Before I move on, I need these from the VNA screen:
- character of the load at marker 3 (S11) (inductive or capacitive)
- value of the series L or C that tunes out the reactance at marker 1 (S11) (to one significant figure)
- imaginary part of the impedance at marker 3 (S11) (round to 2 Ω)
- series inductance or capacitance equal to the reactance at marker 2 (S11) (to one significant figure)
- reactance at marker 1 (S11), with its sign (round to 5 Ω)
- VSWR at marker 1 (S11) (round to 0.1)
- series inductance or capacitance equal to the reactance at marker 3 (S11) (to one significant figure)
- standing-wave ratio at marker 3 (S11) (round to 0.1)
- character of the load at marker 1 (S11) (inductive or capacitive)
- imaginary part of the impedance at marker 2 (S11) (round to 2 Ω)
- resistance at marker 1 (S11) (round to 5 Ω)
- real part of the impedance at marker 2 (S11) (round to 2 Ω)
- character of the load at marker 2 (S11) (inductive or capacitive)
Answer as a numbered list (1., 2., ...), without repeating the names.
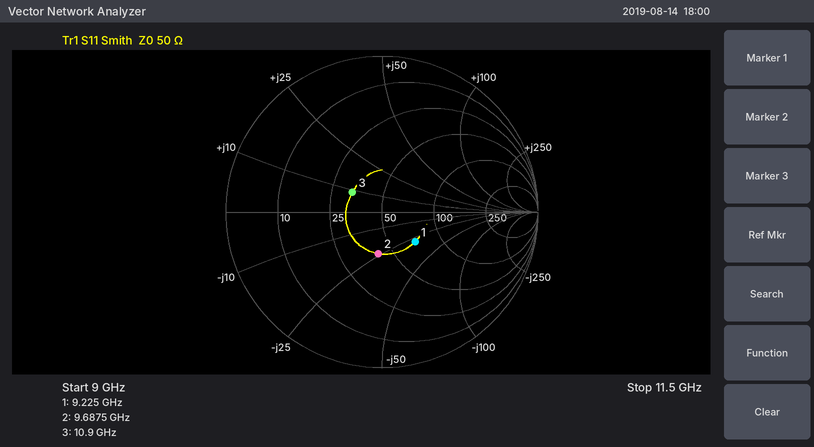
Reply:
1. inductive
2. 500 pH
3. +8 Ω
4. 700 fF
5. -30 Ω
6. 1.8
7. 100 pH
8. 1.6
9. capacitive
10. -24 Ω
11. 70 Ω
12. 42 Ω
13. capacitive
